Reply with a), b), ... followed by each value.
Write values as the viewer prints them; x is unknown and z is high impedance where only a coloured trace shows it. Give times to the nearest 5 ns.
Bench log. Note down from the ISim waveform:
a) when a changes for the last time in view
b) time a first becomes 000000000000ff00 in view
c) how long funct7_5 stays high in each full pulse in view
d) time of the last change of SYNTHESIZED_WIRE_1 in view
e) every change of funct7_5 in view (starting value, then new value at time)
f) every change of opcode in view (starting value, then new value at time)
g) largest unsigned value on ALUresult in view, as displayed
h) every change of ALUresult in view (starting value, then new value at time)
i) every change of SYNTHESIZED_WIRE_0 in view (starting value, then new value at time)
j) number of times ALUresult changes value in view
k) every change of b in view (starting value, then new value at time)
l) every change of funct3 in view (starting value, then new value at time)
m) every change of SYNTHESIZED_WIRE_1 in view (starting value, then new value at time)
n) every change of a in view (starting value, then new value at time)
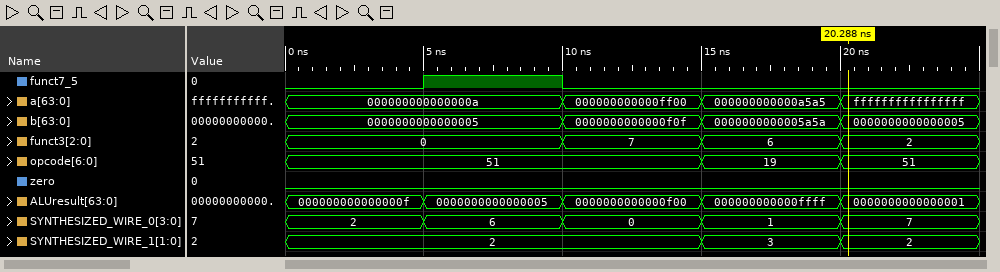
a) 20 ns
b) 10 ns
c) 5 ns
d) 20 ns
e) 0, 1 at 5 ns, 0 at 10 ns
f) 51, 19 at 15 ns, 51 at 20 ns
g) 000000000000ffff
h) 000000000000000f, 0000000000000005 at 5 ns, 0000000000000f00 at 10 ns, 000000000000ffff at 15 ns, 0000000000000001 at 20 ns
i) 2, 6 at 5 ns, 0 at 10 ns, 1 at 15 ns, 7 at 20 ns
j) 4
k) 0000000000000005, 0000000000000f0f at 10 ns, 0000000000005a5a at 15 ns, 0000000000000005 at 20 ns
l) 0, 7 at 10 ns, 6 at 15 ns, 2 at 20 ns
m) 2, 3 at 15 ns, 2 at 20 ns
n) 000000000000000a, 000000000000ff00 at 10 ns, 000000000000a5a5 at 15 ns, ffffffffffffffff at 20 ns
